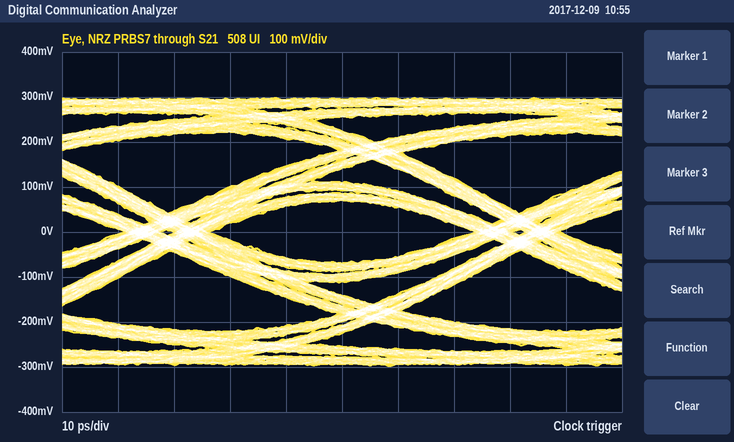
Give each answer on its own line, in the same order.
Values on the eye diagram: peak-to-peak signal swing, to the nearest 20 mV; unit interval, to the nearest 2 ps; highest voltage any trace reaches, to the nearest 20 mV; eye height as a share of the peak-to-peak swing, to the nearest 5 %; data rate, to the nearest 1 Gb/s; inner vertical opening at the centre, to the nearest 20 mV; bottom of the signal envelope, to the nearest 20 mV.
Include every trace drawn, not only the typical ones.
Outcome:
600 mV
62 ps
300 mV
25 %
16 Gb/s
140 mV
-300 mV
